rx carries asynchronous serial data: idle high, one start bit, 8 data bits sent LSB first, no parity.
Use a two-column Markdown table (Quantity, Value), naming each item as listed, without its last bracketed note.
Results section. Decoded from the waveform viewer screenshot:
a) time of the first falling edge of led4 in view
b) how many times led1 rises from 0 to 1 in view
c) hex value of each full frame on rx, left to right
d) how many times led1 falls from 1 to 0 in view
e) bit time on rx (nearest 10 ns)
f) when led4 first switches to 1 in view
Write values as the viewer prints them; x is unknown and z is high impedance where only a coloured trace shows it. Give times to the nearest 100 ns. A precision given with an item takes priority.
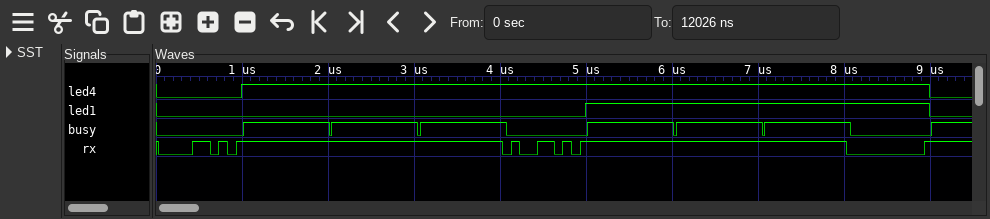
| Quantity | Value |
|---|---|
| time of the first falling edge of led4 in view | 9000 ns |
| how many times led1 rises from 0 to 1 in view | 1 |
| hex value of each full frame on rx, left to right | 58, 59, 00 |
| how many times led1 falls from 1 to 0 in view | 1 |
| bit time on rx | 100 ns |
| when led4 first switches to 1 in view | 1000 ns |
